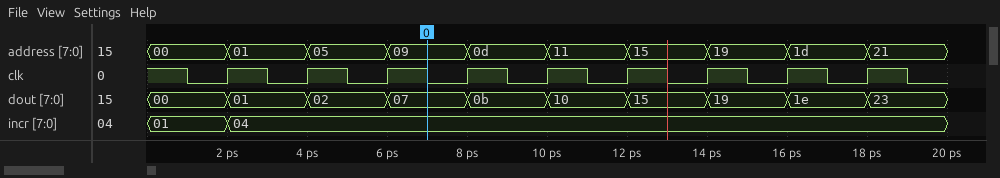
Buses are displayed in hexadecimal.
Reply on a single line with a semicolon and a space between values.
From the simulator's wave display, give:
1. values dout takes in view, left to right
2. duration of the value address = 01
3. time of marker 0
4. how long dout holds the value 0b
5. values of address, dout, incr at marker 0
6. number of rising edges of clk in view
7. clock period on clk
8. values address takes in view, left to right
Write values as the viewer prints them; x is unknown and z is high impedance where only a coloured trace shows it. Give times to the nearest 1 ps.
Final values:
00, 01, 02, 07, 0b, 10, 15, 19, 1e, 23; 2 ps; 7 ps; 2 ps; address=09, dout=07, incr=04; 9; 2 ps; 00, 01, 05, 09, 0d, 11, 15, 19, 1d, 21
